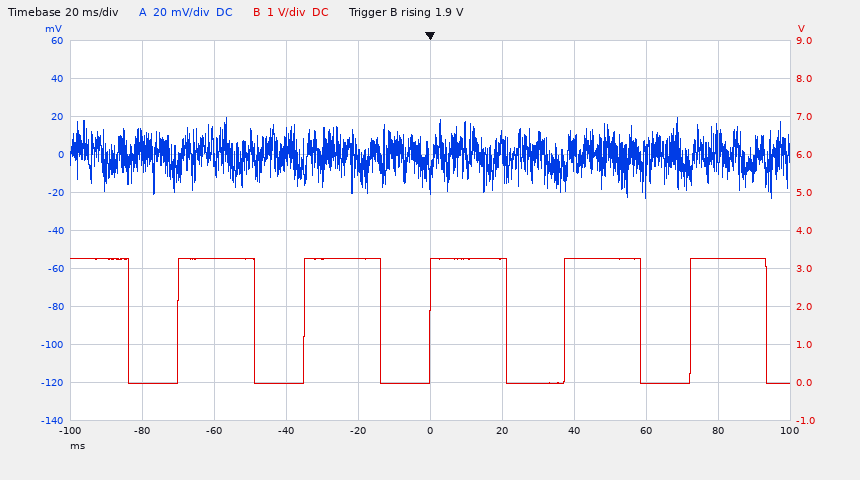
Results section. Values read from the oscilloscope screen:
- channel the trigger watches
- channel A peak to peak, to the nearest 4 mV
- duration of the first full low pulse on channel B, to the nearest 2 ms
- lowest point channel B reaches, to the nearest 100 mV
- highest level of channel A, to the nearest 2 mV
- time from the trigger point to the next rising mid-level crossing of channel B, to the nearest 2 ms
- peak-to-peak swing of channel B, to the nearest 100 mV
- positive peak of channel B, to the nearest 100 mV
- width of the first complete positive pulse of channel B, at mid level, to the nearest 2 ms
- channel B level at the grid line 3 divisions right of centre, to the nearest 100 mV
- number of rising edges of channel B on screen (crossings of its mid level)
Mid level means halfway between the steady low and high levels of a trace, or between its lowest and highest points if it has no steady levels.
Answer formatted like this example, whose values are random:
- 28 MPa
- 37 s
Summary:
- channel B
- 44 mV
- 14 ms
- 0.0 V
- 20 mV
- 38 ms
- 3.3 V
- 3.3 V
- 22 ms
- 0.0 V
- 5
